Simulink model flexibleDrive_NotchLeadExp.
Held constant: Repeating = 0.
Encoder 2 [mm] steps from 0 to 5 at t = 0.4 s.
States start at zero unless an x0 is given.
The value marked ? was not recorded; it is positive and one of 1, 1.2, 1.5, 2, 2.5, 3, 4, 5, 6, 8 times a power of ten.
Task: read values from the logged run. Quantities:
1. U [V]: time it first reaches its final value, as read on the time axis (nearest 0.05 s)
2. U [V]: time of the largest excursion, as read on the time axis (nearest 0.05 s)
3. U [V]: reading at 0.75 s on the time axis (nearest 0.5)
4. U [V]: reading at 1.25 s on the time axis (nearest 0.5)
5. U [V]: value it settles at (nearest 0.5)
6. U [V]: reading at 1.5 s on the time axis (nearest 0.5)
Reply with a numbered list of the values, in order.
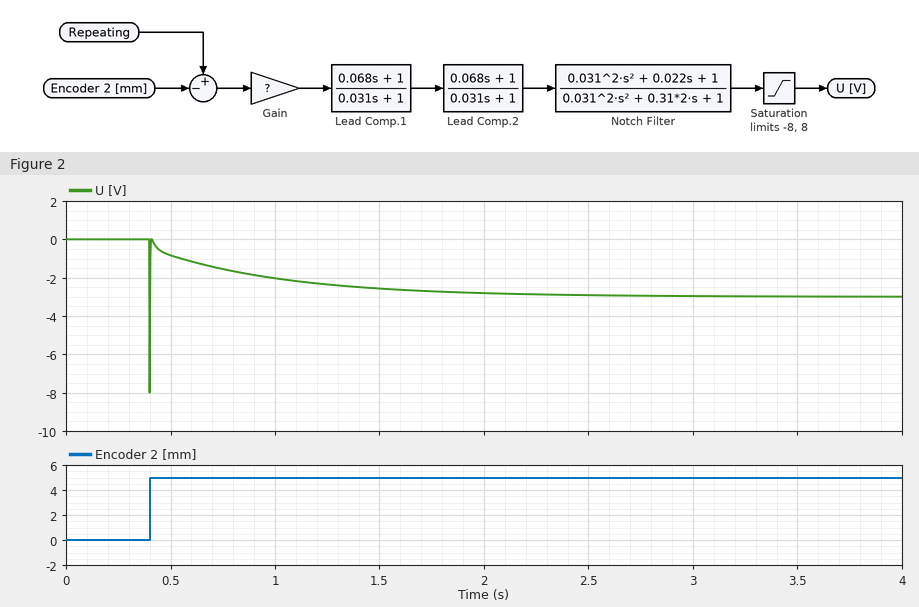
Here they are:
1. 0.40 s
2. 0.40 s
3. -1.5
4. -2.5
5. -3.0
6. -2.5
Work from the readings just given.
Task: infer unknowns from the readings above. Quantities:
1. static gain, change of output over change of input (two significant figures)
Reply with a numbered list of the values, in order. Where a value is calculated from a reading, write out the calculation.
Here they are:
1. (-3 - 0) / (5 - 0) = -0.60
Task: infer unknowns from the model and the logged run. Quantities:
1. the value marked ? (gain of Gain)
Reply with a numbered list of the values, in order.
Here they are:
1. 0.6
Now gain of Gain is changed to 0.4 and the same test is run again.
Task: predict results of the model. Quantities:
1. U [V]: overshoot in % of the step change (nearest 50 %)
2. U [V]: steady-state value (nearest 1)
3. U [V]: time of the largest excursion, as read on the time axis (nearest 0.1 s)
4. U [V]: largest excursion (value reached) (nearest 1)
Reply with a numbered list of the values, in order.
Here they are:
1. 300 %
2. -2
3. 0.4 s
4. -8
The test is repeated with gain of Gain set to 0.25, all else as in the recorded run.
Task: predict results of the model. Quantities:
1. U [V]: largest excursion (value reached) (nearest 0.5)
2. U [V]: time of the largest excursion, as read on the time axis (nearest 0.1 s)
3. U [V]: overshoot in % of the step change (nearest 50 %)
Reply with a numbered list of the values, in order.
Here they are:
1. -6.0
2. 0.4 s
3. 400 %
